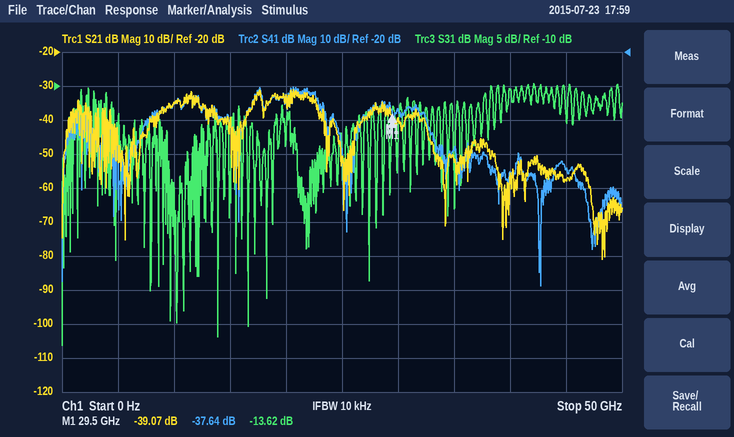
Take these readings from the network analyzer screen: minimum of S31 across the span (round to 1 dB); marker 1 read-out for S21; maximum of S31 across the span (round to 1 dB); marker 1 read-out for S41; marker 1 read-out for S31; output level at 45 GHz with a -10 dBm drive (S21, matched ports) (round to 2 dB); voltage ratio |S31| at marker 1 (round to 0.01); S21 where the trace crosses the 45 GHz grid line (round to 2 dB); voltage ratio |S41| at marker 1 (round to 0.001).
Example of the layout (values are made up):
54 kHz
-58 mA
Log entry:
-48 dB
-39.07 dB
-10 dB
-37.64 dB
-13.62 dB
-68 dBm
0.21
-58 dB
0.013
